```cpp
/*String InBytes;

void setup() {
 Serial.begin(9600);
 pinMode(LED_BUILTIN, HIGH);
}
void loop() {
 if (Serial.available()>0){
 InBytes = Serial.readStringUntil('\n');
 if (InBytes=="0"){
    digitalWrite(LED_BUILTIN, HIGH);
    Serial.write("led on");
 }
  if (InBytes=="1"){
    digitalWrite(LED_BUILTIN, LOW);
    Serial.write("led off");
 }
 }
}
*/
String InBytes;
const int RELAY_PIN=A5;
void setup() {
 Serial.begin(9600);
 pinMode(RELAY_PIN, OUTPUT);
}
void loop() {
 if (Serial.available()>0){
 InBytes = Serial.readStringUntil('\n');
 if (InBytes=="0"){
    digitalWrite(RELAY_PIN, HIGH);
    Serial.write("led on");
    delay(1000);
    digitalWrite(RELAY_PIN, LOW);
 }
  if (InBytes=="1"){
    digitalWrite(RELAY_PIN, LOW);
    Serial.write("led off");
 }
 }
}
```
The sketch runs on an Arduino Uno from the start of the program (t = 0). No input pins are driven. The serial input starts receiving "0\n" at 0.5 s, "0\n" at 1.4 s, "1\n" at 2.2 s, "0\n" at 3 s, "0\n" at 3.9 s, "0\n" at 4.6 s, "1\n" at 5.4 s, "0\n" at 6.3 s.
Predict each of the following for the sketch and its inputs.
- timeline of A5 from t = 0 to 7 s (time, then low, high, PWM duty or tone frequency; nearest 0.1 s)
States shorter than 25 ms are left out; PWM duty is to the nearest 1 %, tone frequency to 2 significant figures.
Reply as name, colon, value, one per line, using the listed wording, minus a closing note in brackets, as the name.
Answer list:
timeline of A5 from t = 0 to 7 s: 0 s low; 0.5 s high; 2.5 s low; 3 s high; 6 s low; 6.3 s high
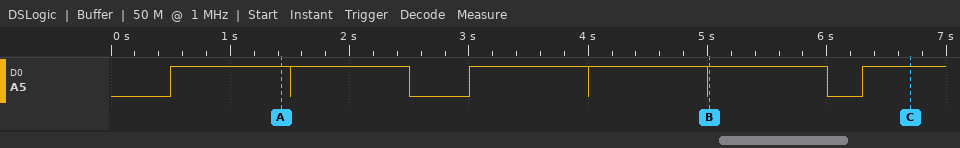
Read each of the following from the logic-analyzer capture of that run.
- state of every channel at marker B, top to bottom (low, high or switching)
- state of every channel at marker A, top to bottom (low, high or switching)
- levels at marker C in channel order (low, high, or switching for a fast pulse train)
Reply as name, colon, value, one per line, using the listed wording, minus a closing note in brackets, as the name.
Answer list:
state of every channel at marker B, top to bottom: A5 high
state of every channel at marker A, top to bottom: A5 high
levels at marker C in channel order: A5 high
